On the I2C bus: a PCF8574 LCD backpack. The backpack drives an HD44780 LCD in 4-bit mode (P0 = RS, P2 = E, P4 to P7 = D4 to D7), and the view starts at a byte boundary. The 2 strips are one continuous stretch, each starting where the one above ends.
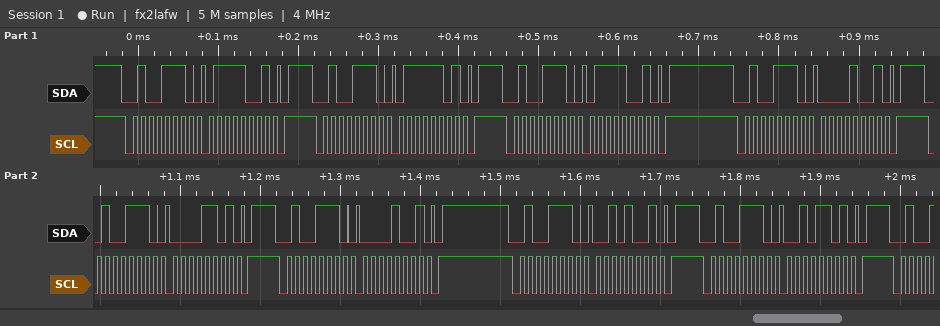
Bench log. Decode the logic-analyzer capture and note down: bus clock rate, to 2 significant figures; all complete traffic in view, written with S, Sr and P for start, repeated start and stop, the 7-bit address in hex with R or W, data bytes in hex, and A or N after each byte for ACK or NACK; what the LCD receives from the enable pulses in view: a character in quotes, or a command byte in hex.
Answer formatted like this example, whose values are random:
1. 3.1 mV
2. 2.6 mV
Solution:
1. 100 kHz
2. S 27W A 79 A P S 27W A 7D A P S 27W A 79 A P S 27W A 09 A P S 27W A 0D A P S 27W A 09 A P S 27W A 29 A P S 27W A 2D A P
3. 'p'
